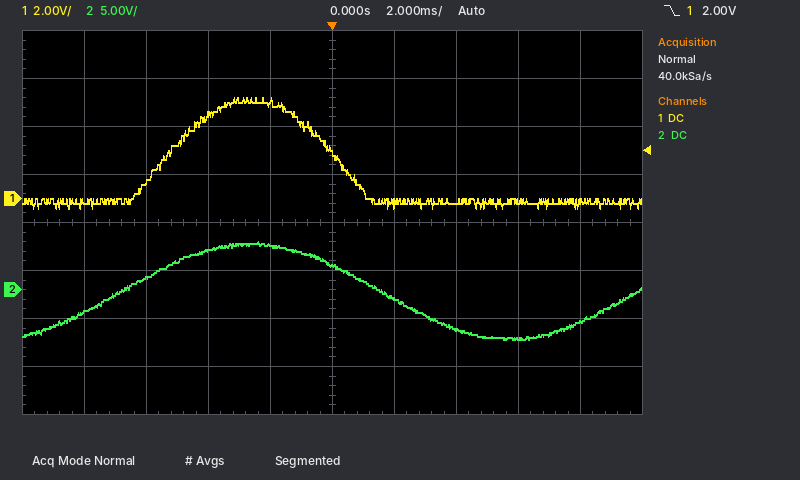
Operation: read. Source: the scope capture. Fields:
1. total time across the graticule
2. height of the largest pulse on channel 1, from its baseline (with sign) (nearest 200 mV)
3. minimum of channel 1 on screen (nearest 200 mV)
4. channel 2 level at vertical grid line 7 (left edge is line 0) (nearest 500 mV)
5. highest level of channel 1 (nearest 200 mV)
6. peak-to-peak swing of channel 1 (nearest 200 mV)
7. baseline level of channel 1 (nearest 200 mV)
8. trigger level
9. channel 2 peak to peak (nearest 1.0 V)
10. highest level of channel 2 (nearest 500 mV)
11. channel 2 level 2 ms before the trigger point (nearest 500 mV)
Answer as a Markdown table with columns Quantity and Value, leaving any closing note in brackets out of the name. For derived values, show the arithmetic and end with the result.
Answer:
| Quantity | Value |
|---|---|
| total time across the graticule | 20 ms |
| height of the largest pulse on channel 1, from its baseline (with sign) | 4.2 V − (-200 mV) = +4.4 V |
| minimum of channel 1 on screen | -400 mV |
| channel 2 level at vertical grid line 7 (left edge is line 0) | -4.0 V |
| highest level of channel 1 | 4.2 V |
| peak-to-peak swing of channel 1 | 4.2 V − (-400 mV) = 4.6 V |
| baseline level of channel 1 | -200 mV |
| trigger level | 2.00 V |
| channel 2 peak to peak | 10.0 V |
| highest level of channel 2 | 5.0 V |
| channel 2 level 2 ms before the trigger point | 4.5 V |
